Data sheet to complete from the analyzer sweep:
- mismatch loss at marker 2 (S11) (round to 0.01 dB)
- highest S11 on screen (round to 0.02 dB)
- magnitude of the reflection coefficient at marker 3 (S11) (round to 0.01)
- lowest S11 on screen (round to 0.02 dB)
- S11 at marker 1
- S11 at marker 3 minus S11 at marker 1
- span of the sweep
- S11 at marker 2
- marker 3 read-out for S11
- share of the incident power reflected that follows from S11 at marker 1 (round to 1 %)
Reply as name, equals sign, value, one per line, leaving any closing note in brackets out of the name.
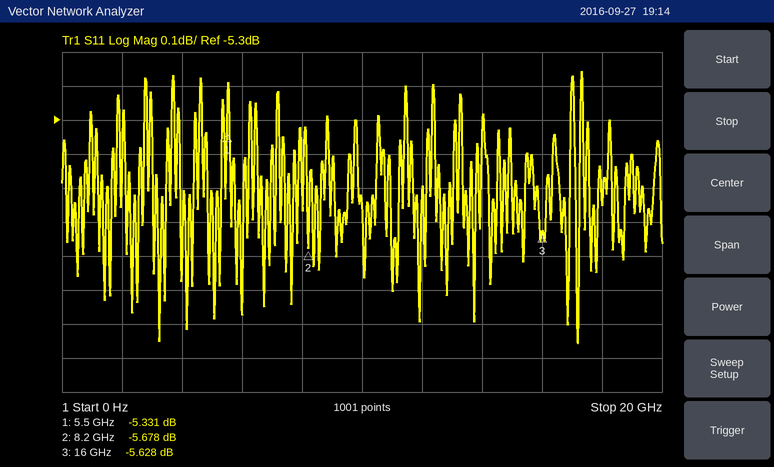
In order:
mismatch loss at marker 2 (S11) = 1.37 dB
highest S11 on screen = -5.16 dB
magnitude of the reflection coefficient at marker 3 (S11) = 0.52
lowest S11 on screen = -5.96 dB
S11 at marker 1 = -5.331 dB
S11 at marker 3 minus S11 at marker 1 = -0.297 dB
span of the sweep = 20 GHz
S11 at marker 2 = -5.678 dB
marker 3 read-out for S11 = -5.628 dB
share of the incident power reflected that follows from S11 at marker 1 = 29 %
